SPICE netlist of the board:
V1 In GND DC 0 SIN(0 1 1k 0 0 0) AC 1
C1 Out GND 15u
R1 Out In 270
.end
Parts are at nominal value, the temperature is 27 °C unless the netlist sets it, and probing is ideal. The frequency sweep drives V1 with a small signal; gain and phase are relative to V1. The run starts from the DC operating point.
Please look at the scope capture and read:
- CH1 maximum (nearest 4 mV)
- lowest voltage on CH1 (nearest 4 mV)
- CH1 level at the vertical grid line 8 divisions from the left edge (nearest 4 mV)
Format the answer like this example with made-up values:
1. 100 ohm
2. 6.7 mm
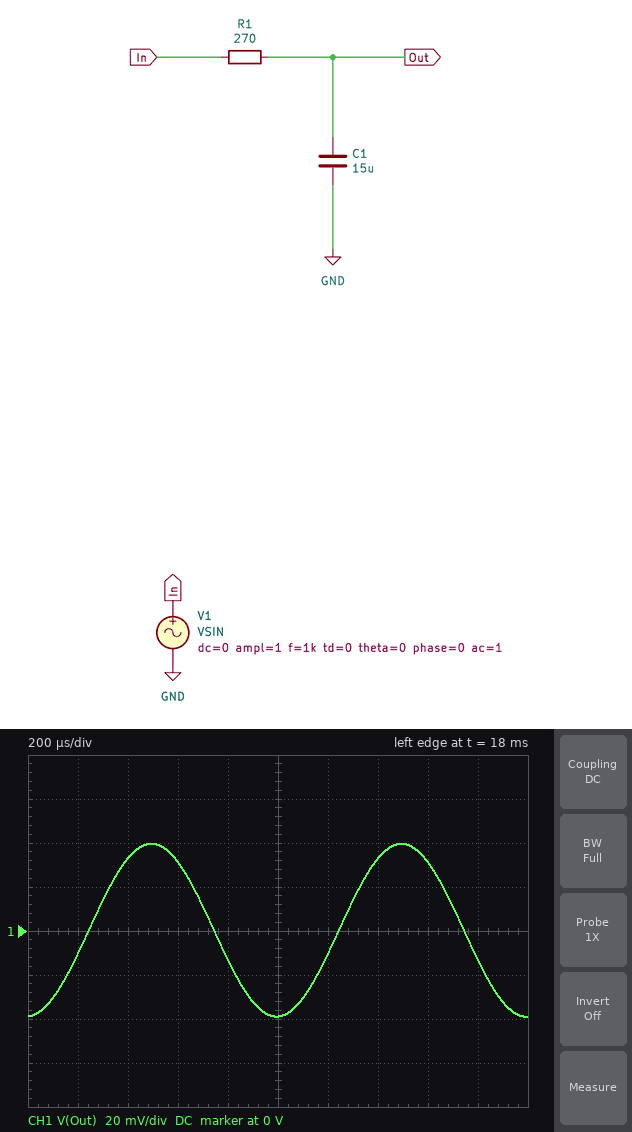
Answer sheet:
1. 40 mV
2. -40 mV
3. 32 mV
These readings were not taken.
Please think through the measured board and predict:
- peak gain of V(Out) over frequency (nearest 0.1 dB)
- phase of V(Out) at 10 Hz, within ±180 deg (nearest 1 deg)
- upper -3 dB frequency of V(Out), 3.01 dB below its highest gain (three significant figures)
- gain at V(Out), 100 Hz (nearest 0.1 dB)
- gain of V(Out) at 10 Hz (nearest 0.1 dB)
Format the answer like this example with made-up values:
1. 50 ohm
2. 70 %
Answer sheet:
1. 0 dB
2. -14 deg
3. 39.3 Hz
4. -8.7 dB
5. -0.3 dB
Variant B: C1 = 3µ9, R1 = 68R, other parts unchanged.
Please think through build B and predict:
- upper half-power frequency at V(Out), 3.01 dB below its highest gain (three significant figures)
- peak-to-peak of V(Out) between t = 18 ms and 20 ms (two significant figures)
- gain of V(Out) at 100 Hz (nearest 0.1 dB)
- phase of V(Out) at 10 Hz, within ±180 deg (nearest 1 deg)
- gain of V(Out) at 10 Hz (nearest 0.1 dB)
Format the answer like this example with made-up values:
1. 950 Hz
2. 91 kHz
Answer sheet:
1. 600 Hz
2. 1.0 V
3. -0.1 dB
4. -1 deg
5. 0 dB
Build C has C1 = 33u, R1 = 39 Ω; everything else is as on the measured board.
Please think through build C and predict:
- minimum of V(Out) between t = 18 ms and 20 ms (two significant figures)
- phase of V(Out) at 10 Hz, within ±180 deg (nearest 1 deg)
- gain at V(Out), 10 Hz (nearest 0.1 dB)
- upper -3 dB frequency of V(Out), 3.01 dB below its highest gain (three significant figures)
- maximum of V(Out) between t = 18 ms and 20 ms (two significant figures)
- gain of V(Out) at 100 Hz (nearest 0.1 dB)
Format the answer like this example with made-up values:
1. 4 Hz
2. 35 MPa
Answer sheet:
1. -120 mV
2. -5 deg
3. 0 dB
4. 124 Hz
5. 120 mV
6. -2.2 dB
